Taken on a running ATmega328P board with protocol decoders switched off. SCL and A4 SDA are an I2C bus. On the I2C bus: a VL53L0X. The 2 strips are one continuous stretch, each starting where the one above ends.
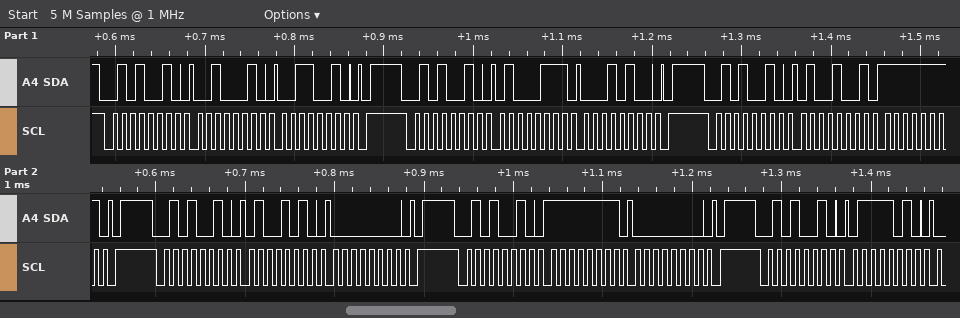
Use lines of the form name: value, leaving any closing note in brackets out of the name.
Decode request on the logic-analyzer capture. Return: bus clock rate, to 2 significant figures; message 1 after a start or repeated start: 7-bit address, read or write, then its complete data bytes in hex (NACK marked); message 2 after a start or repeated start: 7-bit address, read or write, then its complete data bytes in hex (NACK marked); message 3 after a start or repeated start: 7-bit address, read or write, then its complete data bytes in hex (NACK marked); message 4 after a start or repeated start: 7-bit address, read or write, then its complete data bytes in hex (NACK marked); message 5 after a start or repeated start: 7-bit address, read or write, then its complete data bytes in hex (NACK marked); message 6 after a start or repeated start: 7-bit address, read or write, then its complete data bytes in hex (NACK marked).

bus clock rate, to 2 significant figures: 100 kHz
message 1 after a start or repeated start: 7-bit address, read or write, then its complete data bytes in hex: 0x29 write: 22 32
message 2 after a start or repeated start: 7-bit address, read or write, then its complete data bytes in hex: 0x29 write: 47 14
message 3 after a start or repeated start: 7-bit address, read or write, then its complete data bytes in hex: 0x29 write: 49 FF
message 4 after a start or repeated start: 7-bit address, read or write, then its complete data bytes in hex: 0x29 write: 4A 00
message 5 after a start or repeated start: 7-bit address, read or write, then its complete data bytes in hex: 0x29 write: FF 00
message 6 after a start or repeated start: 7-bit address, read or write, then its complete data bytes in hex: 0x29 write: 7A
